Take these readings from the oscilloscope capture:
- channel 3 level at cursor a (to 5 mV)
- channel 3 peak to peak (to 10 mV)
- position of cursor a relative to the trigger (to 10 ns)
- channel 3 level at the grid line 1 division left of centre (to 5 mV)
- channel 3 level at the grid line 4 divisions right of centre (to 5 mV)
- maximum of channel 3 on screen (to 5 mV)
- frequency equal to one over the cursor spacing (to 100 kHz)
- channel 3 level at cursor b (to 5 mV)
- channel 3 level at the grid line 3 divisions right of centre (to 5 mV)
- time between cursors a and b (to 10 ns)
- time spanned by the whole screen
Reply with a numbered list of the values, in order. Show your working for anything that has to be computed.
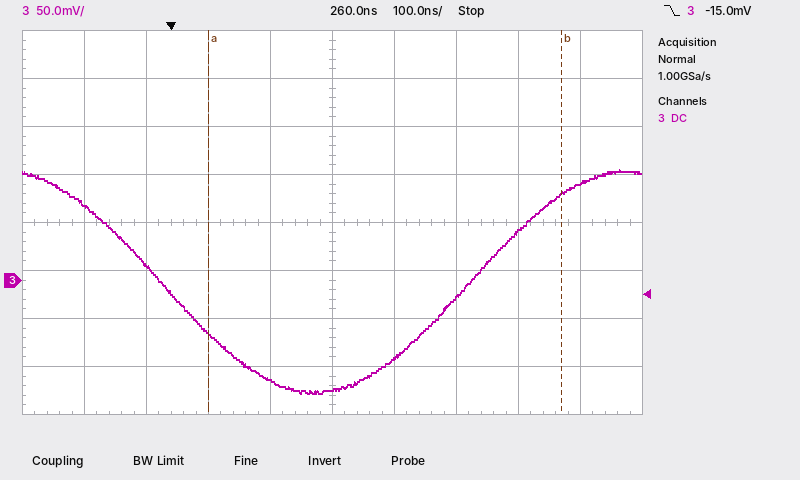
1. -55 mV
2. 230 mV
3. +60 ns
4. -105 mV
5. 100 mV
6. 115 mV
7. 1 / 570 ns ≈ 1.8 MHz
8. 90 mV
9. 50 mV
10. 570 ns
11. 1 µs
